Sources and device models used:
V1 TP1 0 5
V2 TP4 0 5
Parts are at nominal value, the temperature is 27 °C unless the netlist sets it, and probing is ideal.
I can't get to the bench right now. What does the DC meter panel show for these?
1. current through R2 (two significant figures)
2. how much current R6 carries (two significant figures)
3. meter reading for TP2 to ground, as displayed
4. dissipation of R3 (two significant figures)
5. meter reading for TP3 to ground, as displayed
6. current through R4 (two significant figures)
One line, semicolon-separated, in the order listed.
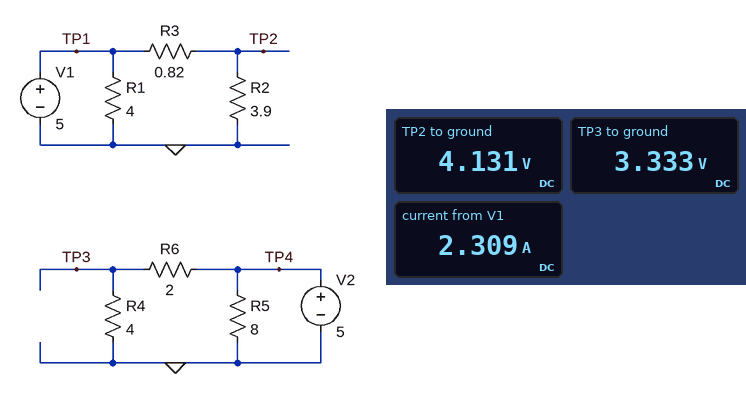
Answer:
1.1 A; 830 mA; 4.131 V; 920 mW; 3.333 V; 830 mA
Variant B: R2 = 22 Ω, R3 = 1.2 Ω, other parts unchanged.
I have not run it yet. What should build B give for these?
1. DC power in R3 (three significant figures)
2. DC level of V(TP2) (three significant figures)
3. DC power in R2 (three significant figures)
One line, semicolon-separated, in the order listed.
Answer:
55.7 mW; 4.74 V; 1.02 W
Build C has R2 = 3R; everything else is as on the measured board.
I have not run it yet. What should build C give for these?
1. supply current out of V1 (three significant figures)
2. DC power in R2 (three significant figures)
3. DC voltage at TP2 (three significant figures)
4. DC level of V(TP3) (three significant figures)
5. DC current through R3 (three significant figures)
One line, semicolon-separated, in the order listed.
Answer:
2.56 A; 5.14 W; 3.93 V; 3.33 V; 1.31 A
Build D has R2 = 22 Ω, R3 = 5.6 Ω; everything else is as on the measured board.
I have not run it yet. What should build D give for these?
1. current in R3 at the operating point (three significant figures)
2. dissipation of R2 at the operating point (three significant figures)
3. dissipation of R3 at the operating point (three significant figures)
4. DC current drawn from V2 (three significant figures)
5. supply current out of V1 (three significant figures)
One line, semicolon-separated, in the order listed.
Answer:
181 mA; 722 mW; 184 mW; 1.46 A; 1.43 A
